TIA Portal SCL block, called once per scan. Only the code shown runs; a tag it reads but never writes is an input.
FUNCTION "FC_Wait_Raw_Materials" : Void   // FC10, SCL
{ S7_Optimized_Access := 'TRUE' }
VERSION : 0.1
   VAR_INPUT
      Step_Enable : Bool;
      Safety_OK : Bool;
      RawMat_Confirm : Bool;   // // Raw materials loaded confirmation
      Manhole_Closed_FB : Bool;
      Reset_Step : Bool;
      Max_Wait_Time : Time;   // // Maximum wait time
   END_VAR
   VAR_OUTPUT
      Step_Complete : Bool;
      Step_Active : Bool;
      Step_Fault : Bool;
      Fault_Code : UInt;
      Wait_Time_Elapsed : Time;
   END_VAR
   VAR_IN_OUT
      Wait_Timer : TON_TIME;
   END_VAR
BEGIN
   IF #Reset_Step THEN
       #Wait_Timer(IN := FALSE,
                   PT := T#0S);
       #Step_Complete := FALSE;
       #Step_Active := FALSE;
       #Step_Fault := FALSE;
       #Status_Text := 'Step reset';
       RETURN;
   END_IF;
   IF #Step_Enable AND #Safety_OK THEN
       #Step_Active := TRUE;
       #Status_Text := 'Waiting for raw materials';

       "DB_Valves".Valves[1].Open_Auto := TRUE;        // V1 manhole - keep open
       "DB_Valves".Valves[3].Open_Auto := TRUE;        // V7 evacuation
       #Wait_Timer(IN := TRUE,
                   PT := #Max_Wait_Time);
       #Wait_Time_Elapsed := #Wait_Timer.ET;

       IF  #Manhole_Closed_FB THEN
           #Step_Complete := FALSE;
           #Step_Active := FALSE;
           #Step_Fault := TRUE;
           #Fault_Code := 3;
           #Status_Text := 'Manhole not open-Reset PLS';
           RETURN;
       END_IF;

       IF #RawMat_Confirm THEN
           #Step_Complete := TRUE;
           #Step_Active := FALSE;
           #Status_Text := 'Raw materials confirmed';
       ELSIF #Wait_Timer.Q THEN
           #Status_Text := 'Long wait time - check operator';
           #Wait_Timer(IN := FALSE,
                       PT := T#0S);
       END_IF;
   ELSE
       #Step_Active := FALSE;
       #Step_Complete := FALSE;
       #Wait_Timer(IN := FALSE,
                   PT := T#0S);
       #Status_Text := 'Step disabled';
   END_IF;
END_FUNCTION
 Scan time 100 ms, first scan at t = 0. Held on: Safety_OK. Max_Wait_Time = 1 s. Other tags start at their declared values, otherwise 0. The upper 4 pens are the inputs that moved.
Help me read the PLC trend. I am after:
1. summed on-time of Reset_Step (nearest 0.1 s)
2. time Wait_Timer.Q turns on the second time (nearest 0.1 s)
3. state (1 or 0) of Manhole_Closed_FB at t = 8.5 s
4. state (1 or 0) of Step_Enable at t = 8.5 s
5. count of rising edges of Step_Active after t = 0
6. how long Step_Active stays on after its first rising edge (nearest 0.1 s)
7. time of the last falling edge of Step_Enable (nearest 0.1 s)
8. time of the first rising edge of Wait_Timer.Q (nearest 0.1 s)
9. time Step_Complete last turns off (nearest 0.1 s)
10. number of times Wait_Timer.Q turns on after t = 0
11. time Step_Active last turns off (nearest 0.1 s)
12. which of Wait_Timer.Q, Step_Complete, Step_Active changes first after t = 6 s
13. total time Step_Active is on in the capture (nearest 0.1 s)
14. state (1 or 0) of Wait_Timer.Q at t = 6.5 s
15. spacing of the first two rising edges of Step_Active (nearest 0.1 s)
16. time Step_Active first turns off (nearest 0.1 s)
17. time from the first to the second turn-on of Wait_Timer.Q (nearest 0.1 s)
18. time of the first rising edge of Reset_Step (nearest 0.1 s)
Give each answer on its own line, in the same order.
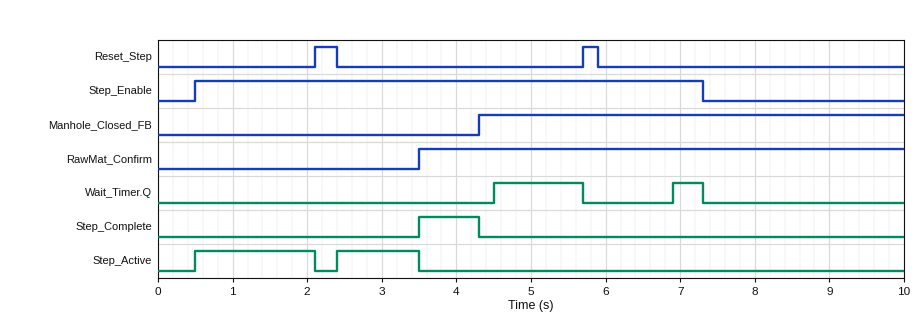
0.5 s
6.9 s
1
0
2
1.6 s
7.3 s
4.5 s
4.3 s
2
3.5 s
Wait_Timer.Q
2.7 s
0
1.9 s
2.1 s
2.4 s
2.1 s
